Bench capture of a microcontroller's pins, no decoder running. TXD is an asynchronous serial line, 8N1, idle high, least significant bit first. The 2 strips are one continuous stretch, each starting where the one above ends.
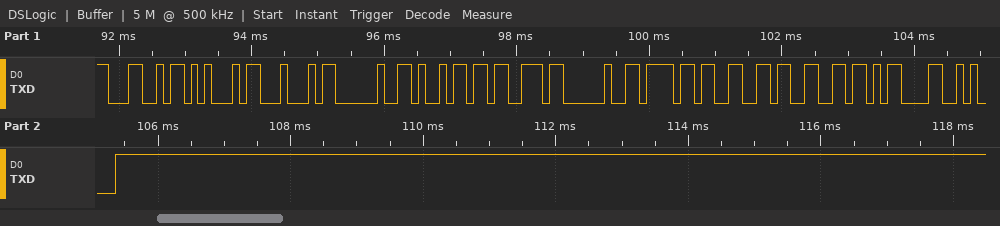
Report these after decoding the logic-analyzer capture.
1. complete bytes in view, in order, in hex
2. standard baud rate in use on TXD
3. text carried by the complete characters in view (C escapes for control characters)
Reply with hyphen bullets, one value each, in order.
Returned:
- 4C 45 44 20 69 73 20 6F 66 66 0D 0A
- 9600 baud
- "LED is off\r\n"
